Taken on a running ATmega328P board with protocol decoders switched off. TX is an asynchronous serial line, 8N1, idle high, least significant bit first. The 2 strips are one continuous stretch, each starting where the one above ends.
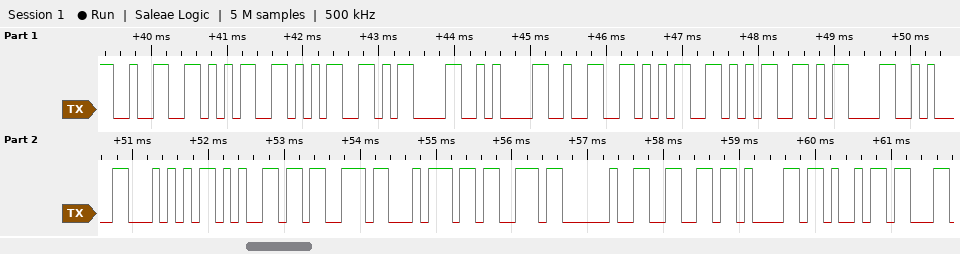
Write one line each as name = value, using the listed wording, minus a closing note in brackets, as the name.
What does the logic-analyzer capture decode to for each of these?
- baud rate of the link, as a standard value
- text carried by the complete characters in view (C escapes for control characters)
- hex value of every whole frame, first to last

baud rate of the link, as a standard value = 9600 baud
text carried by the complete characters in view = "255\r\n255\r\nTests fai"
hex value of every whole frame, first to last = 32 35 35 0D 0A 32 35 35 0D 0A 54 65 73 74 73 20 66 61 69
